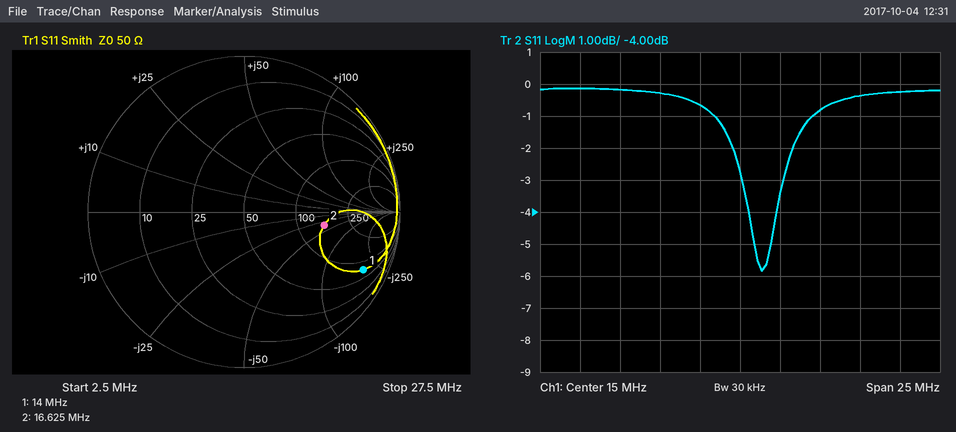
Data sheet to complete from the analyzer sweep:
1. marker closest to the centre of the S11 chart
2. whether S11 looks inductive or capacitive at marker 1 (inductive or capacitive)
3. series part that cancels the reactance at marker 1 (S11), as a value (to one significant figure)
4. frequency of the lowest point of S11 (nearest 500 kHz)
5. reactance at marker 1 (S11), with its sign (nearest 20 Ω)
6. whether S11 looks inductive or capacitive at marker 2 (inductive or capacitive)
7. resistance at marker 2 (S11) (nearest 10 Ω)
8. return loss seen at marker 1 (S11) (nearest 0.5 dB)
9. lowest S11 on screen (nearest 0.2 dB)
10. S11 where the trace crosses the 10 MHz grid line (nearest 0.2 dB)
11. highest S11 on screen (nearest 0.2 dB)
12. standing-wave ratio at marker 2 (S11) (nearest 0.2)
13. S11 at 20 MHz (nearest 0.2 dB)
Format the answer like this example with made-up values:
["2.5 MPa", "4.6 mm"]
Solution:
["marker 2", "capacitive", "2 µH", "16.5 MHz", "-200 Ω", "capacitive", "150 Ω", "1.5 dB", "-5.8 dB", "-0.2 dB", "-0.2 dB", "3.2", "-0.8 dB"]
